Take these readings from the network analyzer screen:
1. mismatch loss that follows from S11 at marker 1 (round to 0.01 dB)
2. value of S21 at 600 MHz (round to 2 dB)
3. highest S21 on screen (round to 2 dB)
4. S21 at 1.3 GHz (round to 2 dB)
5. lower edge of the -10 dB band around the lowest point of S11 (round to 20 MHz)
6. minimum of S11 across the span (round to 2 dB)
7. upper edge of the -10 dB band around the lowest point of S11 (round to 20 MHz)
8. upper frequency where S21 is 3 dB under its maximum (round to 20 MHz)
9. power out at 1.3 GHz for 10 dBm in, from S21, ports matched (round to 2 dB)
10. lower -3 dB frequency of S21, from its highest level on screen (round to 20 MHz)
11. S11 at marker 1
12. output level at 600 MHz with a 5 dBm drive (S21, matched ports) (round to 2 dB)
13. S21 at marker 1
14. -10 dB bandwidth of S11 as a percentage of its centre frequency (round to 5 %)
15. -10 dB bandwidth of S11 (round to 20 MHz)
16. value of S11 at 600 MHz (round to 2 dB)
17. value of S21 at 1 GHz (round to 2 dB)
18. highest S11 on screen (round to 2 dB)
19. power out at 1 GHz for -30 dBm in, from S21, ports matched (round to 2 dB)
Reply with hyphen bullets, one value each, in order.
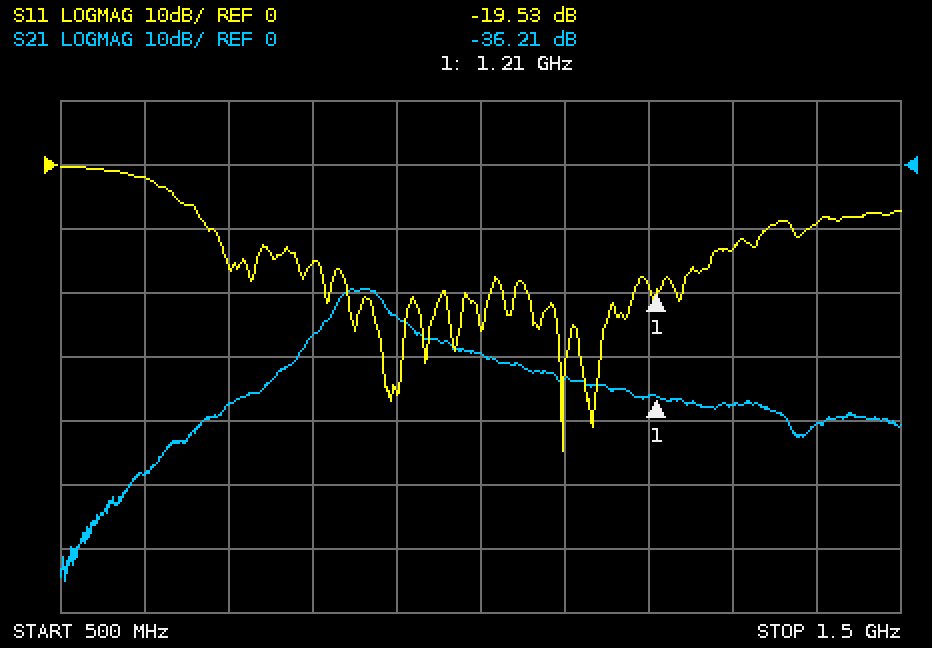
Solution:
- 0.05 dB
- -48 dB
- -20 dB
- -38 dB
- 680 MHz
- -44 dB
- 1.34 GHz
- 880 MHz
- -28 dBm
- 820 MHz
- -19.53 dB
- -44 dBm
- -36.21 dB
- 65 %
- 660 MHz
- -2 dB
- -30 dB
- 0 dB
- -60 dBm
